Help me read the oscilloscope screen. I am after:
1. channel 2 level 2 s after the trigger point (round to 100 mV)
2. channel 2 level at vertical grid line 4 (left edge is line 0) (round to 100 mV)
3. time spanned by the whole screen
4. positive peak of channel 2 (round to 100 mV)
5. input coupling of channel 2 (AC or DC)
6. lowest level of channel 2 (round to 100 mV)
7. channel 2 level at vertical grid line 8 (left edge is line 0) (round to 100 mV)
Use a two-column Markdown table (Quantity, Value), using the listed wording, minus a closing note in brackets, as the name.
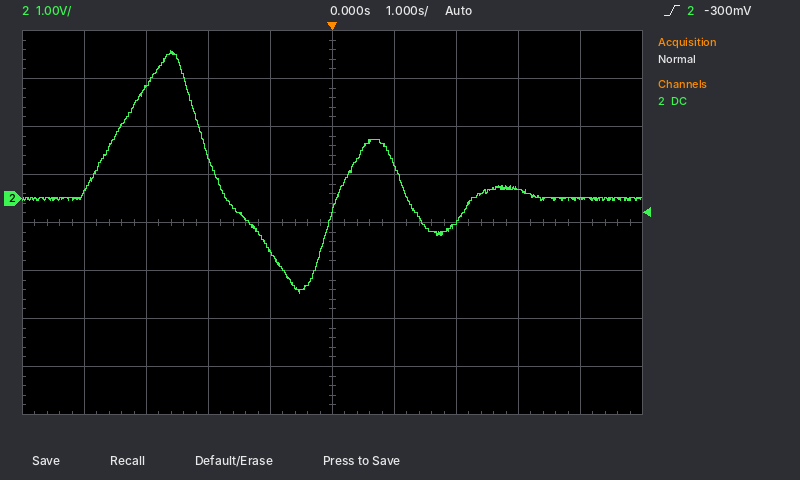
| Quantity | Value |
|---|---|
| channel 2 level 2 s after the trigger point | -500 mV |
| channel 2 level at vertical grid line 4 (left edge is line 0) | -1.1 V |
| time spanned by the whole screen | 10 s |
| positive peak of channel 2 | 3.1 V |
| input coupling of channel 2 | DC |
| lowest level of channel 2 | -2.0 V |
| channel 2 level at vertical grid line 8 (left edge is line 0) | 200 mV |
